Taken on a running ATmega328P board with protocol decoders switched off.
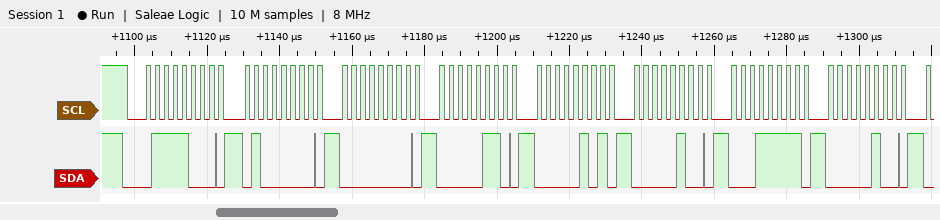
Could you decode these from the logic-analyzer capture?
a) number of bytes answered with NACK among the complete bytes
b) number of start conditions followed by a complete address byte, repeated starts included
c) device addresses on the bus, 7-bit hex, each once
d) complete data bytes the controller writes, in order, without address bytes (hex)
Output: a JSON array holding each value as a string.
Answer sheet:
["0", "1", "0x3C", "40 00 06 05 04 1F 04"]
